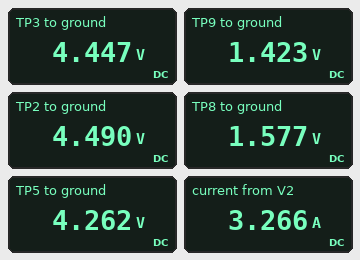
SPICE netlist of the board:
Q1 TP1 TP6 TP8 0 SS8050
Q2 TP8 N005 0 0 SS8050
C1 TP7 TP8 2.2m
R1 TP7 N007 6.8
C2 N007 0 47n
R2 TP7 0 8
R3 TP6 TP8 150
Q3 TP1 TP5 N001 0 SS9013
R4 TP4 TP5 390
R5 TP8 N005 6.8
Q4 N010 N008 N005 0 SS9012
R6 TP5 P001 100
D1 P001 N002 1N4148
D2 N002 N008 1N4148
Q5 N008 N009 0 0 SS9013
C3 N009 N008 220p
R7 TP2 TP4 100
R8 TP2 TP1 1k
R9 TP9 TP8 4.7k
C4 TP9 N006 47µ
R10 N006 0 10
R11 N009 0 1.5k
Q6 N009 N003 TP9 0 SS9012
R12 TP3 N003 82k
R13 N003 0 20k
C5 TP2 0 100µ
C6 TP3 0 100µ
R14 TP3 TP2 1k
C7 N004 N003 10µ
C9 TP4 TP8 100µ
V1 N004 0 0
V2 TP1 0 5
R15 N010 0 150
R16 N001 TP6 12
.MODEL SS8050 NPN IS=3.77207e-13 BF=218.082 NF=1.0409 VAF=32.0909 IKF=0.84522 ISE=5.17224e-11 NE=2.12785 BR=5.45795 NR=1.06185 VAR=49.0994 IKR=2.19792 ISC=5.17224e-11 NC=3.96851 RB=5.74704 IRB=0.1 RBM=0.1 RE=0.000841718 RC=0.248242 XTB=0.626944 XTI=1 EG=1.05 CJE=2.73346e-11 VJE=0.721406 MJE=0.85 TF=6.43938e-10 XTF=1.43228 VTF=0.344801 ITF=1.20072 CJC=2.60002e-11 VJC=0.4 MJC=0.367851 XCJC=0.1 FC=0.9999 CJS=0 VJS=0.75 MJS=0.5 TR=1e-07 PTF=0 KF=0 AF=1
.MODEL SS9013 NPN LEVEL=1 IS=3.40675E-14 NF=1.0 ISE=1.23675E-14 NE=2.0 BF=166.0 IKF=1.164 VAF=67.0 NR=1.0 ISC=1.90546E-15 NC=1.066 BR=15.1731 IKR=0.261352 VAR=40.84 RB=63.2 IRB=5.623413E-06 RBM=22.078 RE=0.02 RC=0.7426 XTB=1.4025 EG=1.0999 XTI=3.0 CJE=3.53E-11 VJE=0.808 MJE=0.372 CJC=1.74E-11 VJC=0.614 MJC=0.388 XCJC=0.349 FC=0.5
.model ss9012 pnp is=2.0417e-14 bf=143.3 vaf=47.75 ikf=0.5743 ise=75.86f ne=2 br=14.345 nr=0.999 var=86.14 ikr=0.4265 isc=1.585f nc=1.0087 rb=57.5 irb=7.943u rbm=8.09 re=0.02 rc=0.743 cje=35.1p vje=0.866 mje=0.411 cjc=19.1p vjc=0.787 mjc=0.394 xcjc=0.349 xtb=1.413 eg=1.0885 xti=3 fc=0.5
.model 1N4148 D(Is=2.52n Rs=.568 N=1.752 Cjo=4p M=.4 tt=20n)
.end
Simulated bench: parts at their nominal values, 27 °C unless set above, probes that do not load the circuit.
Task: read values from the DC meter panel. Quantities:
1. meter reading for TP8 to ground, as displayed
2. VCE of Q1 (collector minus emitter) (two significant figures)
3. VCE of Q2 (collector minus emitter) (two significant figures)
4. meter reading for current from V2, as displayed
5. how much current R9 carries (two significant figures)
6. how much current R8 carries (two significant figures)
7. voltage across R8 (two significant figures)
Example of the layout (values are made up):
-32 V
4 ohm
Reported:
1.577 V
3.4 V
1.6 V
3.266 A
33 µA
510 µA
510 mV
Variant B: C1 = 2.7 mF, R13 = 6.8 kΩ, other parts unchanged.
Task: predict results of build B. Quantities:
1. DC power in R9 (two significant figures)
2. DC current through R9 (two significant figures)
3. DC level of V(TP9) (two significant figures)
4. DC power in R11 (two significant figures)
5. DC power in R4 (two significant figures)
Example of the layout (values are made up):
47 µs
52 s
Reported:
88 µW
140 µA
930 mV
28 µW
84 µW
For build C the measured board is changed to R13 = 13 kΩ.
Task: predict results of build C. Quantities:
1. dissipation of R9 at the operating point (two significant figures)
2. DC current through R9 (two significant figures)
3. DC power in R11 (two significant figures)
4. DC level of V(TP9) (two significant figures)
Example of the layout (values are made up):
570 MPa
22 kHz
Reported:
32 µW
83 µA
10 µW
1.2 V
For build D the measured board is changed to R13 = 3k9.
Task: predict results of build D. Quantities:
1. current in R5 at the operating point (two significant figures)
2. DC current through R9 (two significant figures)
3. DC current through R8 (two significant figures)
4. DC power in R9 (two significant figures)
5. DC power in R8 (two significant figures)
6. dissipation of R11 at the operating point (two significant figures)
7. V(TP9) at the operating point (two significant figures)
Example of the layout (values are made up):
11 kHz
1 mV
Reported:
72 mA
170 µA
520 µA
130 µW
270 µW
41 µW
800 mV
